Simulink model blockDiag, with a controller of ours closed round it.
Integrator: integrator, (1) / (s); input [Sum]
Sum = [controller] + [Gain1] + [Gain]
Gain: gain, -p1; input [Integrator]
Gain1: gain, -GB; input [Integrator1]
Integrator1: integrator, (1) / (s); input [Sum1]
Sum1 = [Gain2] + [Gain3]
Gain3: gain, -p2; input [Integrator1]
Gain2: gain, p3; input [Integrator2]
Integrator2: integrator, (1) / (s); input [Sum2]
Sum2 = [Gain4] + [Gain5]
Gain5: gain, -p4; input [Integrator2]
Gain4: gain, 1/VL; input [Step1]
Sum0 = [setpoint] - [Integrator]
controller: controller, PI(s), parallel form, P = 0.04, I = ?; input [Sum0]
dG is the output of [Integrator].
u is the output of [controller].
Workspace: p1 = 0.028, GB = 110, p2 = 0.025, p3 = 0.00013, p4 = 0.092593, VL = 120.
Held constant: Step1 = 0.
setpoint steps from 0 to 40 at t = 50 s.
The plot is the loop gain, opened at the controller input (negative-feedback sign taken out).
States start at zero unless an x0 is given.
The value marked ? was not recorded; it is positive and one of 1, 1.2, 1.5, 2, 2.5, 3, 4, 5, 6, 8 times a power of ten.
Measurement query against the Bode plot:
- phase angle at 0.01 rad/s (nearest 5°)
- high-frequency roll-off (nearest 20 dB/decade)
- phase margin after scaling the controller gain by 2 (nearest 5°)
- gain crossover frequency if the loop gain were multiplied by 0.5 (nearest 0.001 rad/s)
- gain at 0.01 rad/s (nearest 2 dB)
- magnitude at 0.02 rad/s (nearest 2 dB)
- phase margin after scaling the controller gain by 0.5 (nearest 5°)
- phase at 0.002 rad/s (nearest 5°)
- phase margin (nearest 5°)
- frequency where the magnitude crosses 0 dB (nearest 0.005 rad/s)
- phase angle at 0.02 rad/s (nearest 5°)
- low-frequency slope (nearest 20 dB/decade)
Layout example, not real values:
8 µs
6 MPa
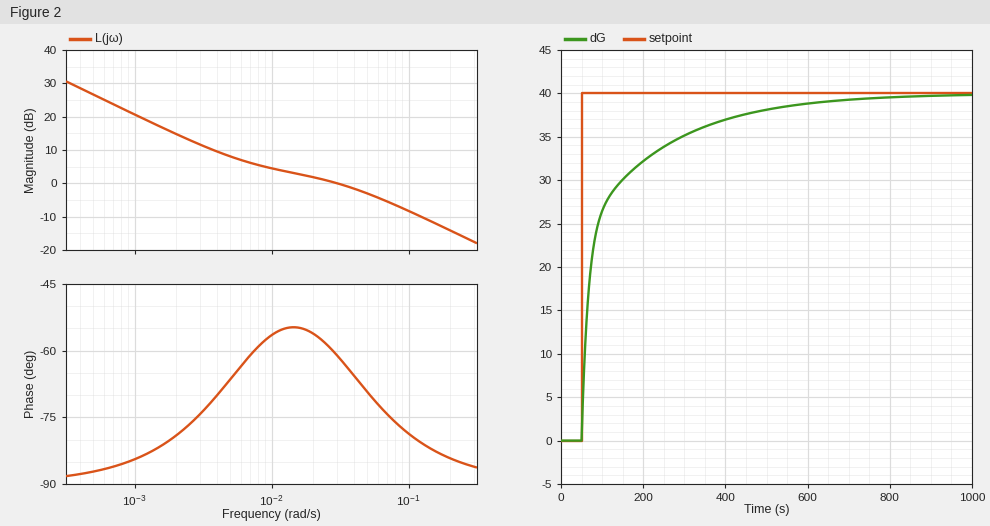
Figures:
-55°
-20 dB/decade
105°
0.007 rad/s
4 dB
2 dB
120°
-80°
120°
0.030 rad/s
-55°
-20 dB/decade
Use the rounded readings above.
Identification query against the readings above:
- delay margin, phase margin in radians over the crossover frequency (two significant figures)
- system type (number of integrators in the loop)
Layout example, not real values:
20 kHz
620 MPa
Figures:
70 s
1
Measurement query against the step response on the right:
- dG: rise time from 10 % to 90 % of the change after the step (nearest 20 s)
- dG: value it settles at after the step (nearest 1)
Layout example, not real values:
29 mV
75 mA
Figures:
280 s
40
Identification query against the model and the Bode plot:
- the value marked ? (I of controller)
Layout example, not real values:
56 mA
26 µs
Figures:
0.0003
